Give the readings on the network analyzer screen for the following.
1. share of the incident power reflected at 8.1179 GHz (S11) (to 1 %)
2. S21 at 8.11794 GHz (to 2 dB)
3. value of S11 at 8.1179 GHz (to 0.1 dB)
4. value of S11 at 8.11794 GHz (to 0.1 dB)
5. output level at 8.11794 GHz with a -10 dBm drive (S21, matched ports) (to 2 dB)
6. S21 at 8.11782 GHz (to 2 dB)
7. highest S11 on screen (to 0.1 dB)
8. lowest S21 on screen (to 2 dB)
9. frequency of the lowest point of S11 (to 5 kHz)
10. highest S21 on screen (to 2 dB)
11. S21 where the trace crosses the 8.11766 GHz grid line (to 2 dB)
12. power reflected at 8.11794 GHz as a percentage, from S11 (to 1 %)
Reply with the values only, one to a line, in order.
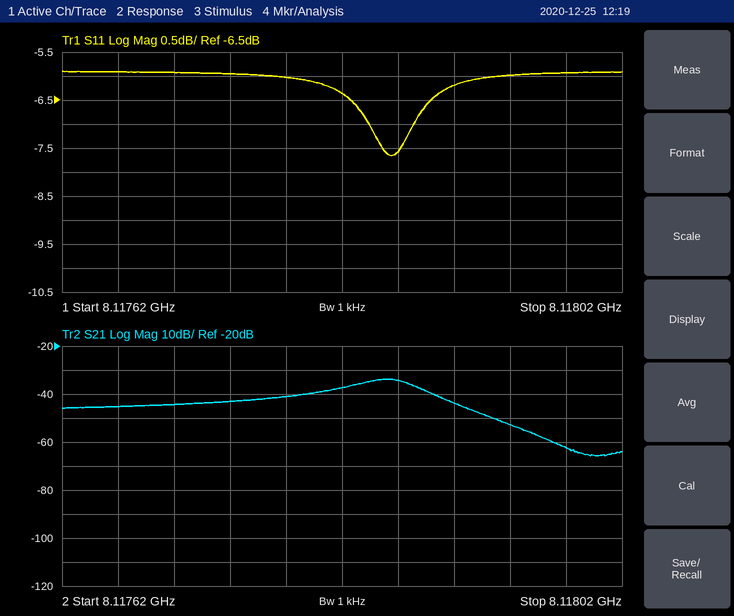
24 %
-52 dB
-6.2 dB
-6.0 dB
-62 dBm
-38 dB
-5.9 dB
-66 dB
8.117855 GHz
-34 dB
-46 dB
25 %
